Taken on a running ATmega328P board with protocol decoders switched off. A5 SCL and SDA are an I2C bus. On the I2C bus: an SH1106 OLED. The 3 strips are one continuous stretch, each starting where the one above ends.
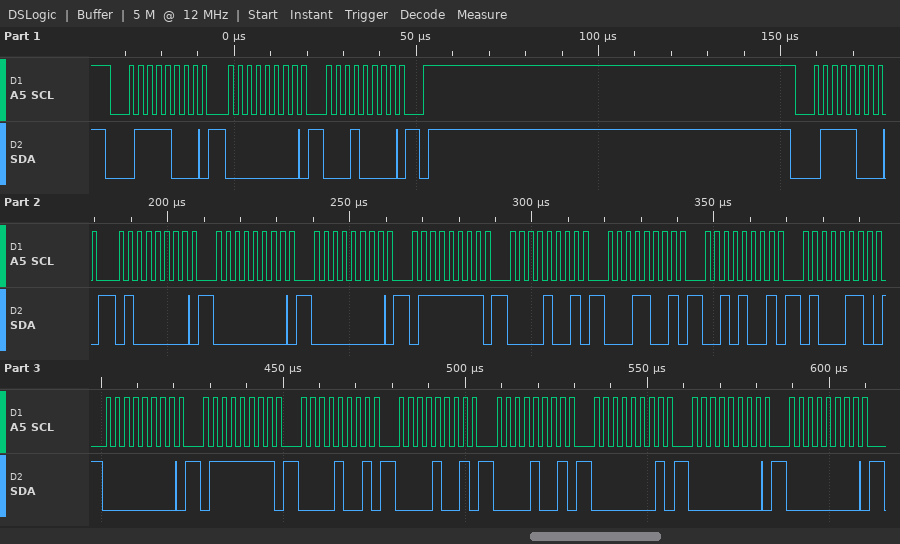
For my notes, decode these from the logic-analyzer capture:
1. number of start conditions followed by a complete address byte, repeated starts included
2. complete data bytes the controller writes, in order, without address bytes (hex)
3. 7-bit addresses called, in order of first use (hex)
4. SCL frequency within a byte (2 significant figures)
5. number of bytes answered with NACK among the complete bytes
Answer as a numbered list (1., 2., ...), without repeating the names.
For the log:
1. 2
2. 00 10 40 00 00 7F 09 19 29 46 00 7F 09 09 09 01 00 00
3. 0x3C
4. 400 kHz
5. 0
